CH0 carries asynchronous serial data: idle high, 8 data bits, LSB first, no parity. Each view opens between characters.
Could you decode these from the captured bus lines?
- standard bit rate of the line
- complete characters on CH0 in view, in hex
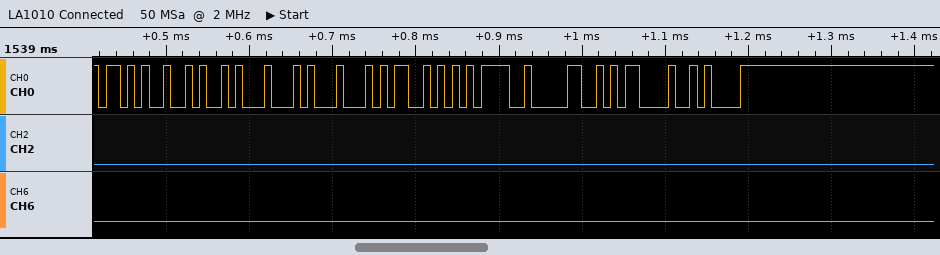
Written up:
115200 baud
2B, 4A, 44, 44, 53, 3D, 30, 0D, 0A
